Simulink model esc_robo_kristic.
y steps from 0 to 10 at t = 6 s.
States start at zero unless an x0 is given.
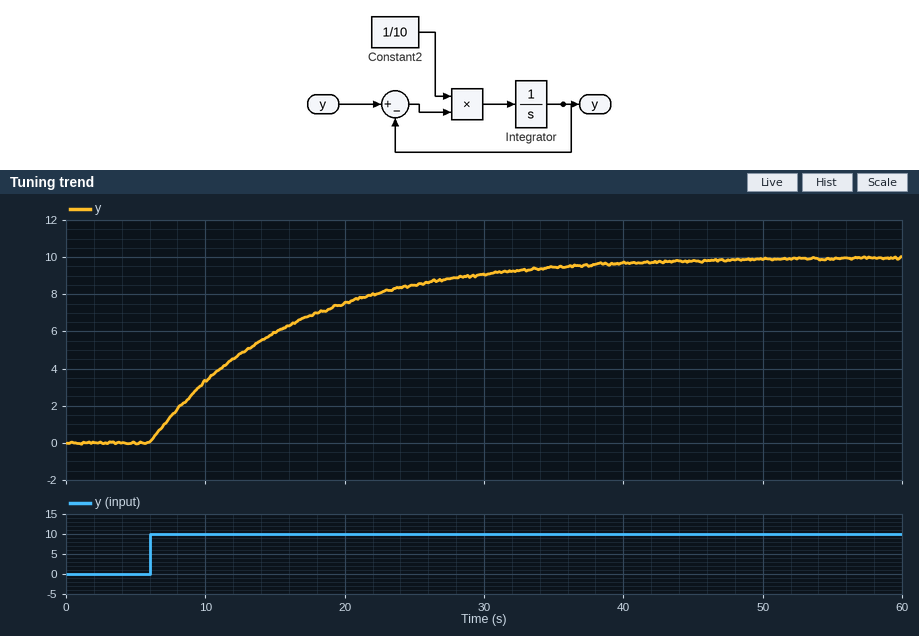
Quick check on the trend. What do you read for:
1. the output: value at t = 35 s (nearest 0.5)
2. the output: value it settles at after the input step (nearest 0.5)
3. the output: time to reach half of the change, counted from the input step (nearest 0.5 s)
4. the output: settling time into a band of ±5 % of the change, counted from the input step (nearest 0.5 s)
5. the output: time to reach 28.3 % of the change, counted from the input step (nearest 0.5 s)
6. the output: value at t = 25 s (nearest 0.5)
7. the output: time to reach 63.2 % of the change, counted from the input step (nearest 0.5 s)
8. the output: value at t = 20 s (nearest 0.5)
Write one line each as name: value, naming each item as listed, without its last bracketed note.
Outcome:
the output: value at t = 35 s: 9.5
the output: value it settles at after the input step: 10.0
the output: time to reach half of the change, counted from the input step: 7.0 s
the output: settling time into a band of ±5 % of the change, counted from the input step: 30.0 s
the output: time to reach 28.3 % of the change, counted from the input step: 3.5 s
the output: value at t = 25 s: 8.5
the output: time to reach 63.2 % of the change, counted from the input step: 10.0 s
the output: value at t = 20 s: 7.5
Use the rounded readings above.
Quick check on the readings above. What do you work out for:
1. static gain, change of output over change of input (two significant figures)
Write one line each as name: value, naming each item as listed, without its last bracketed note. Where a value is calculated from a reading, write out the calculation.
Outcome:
static gain, change of output over change of input: (10 - 0) / (10 - 0) = 1.0
